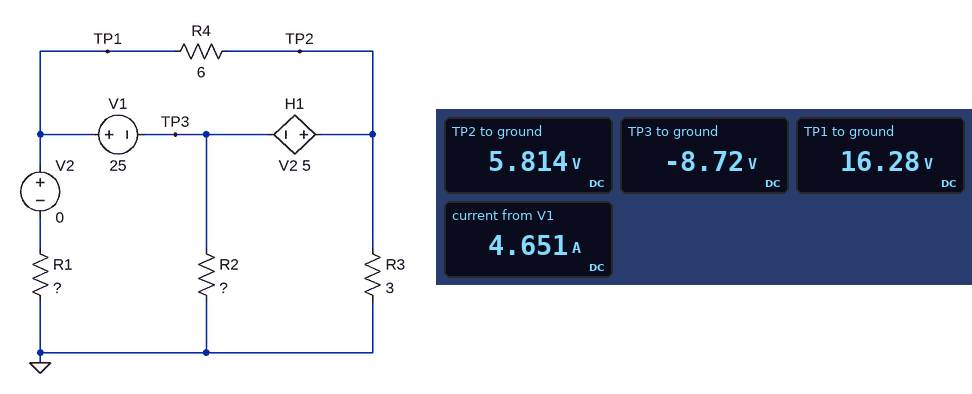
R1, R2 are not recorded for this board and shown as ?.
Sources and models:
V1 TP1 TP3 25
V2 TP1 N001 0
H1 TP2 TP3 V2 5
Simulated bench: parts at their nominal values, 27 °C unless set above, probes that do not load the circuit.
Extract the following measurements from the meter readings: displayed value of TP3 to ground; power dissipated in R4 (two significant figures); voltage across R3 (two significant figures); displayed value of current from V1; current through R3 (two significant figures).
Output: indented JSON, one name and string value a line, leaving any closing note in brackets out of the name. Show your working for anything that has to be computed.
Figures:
{
  "displayed value of TP3 to ground": "-8.72 V",
  "power dissipated in R4": "(16.28 V - 5.814 V)^2 / 6 Ω = 18 W",
  "voltage across R3": "5.814 V = 5.8 V",
  "displayed value of current from V1": "4.651 A",
  "current through R3": "(5.814 V) / 3 Ω = 1.9 A"
}
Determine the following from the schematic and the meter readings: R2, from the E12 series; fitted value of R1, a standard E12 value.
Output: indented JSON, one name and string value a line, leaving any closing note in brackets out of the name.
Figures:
{
  "R2, from the E12 series": "1.8 Ω",
  "fitted value of R1, a standard E12 value": "5.6 Ω"
}
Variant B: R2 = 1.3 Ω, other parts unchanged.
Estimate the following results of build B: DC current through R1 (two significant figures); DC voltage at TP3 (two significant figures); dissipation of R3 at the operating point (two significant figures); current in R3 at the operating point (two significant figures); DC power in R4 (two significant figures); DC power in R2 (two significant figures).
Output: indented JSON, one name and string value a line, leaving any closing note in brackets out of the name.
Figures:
{
  "DC current through R1": "3.1 A",
  "DC voltage at TP3": "-7.5 V",
  "dissipation of R3 at the operating point": "22 W",
  "current in R3 at the operating point": "2.7 A",
  "DC power in R4": "15 W",
  "DC power in R2": "44 W"
}
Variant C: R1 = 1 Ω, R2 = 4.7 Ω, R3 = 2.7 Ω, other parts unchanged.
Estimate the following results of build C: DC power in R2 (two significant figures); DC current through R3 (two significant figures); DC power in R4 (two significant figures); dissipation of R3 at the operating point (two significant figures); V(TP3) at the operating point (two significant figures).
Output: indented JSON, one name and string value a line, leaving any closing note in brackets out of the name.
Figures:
{
  "DC power in R2": "92 W",
  "DC current through R3": "170 mA",
  "DC power in R4": "2.4 W",
  "dissipation of R3 at the operating point": "80 mW",
  "V(TP3) at the operating point": "-21 V"
}
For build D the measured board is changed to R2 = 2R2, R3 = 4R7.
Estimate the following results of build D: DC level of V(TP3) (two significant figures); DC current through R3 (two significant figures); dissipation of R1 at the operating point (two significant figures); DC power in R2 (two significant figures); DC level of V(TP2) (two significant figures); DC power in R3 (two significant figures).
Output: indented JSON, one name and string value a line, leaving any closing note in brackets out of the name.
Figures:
{
  "DC level of V(TP3)": "-8.9 V",
  "DC current through R3": "1.2 A",
  "dissipation of R1 at the operating point": "46 W",
  "DC power in R2": "36 W",
  "DC level of V(TP2)": "5.5 V",
  "DC power in R3": "6.4 W"
}
